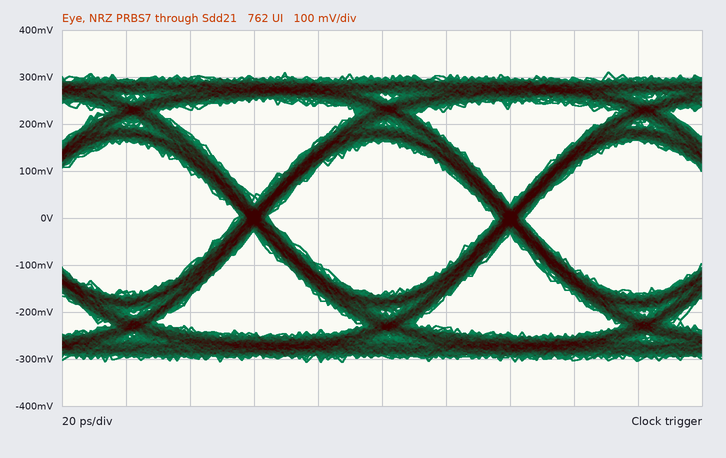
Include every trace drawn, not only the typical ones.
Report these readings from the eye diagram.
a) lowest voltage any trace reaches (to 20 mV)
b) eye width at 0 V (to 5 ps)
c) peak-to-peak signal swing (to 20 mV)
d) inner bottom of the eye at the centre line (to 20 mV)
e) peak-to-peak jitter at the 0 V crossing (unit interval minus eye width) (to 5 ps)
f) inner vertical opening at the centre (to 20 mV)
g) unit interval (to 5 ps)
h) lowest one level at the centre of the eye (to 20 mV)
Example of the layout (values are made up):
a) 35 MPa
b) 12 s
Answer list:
a) -300 mV
b) 70 ps
c) 620 mV
d) -160 mV
e) 10 ps
f) 320 mV
g) 80 ps
h) 160 mV
